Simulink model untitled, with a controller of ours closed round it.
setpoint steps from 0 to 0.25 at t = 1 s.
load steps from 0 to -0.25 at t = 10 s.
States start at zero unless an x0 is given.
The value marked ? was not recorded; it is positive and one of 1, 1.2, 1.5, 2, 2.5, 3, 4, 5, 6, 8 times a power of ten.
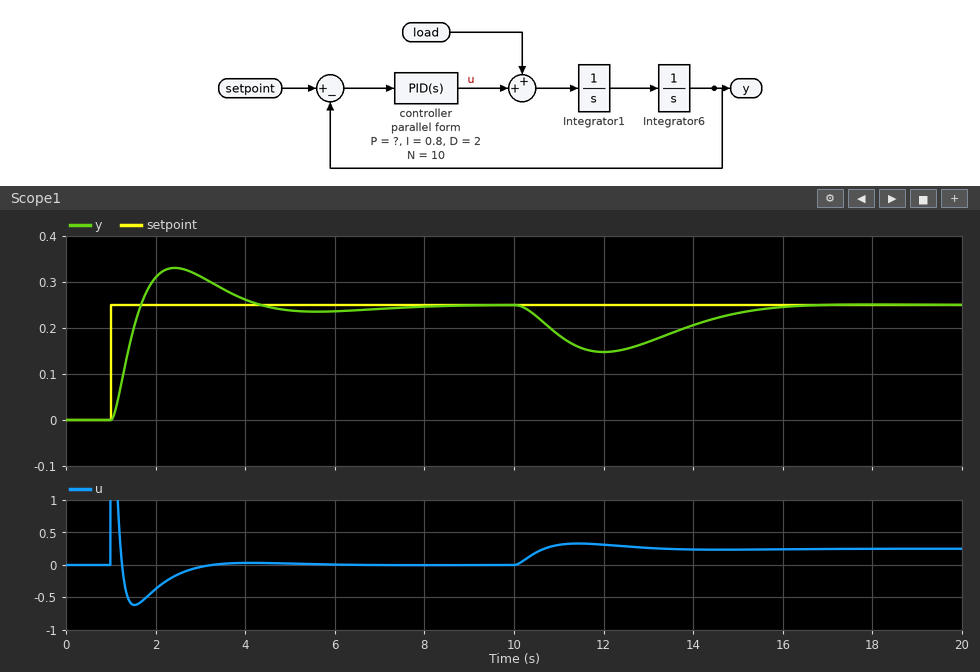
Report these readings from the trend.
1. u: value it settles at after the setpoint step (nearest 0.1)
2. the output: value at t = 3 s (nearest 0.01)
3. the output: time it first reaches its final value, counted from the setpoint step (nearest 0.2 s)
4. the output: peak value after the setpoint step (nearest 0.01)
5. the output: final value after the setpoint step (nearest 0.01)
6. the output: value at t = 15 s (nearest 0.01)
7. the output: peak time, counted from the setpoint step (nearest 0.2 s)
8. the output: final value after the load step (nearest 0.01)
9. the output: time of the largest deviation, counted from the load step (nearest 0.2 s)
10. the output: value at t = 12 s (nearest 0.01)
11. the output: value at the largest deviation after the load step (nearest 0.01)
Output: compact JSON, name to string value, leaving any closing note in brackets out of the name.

{"u: value it settles at after the setpoint step": "0.0", "the output: value at t = 3 s": "0.31", "the output: time it first reaches its final value, counted from the setpoint step": "0.6 s", "the output: peak value after the setpoint step": "0.33", "the output: final value after the setpoint step": "0.25", "the output: value at t = 15 s": "0.23", "the output: peak time, counted from the setpoint step": "1.4 s", "the output: final value after the load step": "0.25", "the output: time of the largest deviation, counted from the load step": "2.0 s", "the output: value at t = 12 s": "0.15", "the output: value at the largest deviation after the load step": "0.15"}
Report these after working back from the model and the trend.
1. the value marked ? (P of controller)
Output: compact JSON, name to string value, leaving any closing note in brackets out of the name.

{"the value marked ?": "2"}
